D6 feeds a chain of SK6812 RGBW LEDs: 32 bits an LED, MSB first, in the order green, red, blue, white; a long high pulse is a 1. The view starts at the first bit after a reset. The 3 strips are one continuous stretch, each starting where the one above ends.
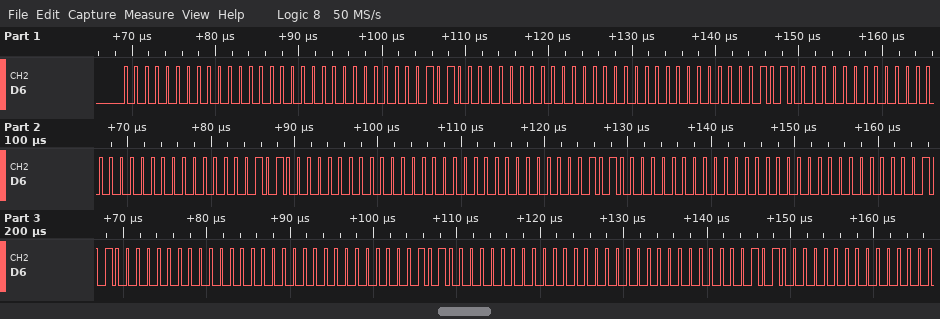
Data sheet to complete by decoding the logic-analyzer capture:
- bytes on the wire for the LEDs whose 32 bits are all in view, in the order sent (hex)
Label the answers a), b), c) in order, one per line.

a) 00 00 00 05 00 00 00 05 00 00 00 05 00 00 00 05 00 00 00 05 00 00 00 05 00 00 00 05
